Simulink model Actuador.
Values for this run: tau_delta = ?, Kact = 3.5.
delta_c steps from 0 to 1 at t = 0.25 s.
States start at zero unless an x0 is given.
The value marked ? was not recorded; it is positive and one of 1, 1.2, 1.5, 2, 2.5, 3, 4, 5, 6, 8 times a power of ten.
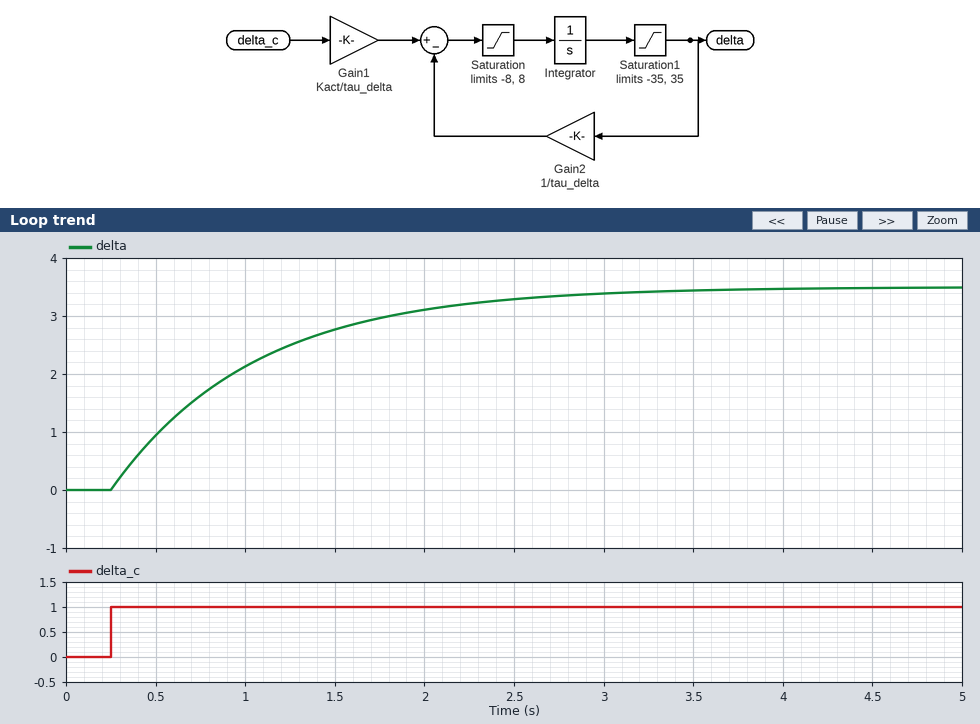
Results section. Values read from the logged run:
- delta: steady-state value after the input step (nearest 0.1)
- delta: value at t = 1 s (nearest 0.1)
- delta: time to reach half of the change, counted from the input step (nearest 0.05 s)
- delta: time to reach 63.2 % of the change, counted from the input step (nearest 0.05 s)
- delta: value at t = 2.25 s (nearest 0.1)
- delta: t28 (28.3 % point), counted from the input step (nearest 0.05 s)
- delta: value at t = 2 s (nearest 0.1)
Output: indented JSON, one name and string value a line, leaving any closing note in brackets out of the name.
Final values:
{
  "delta: steady-state value after the input step": "3.5",
  "delta: value at t = 1 s": "2.1",
  "delta: time to reach half of the change, counted from the input step": "0.55 s",
  "delta: time to reach 63.2 % of the change, counted from the input step": "0.80 s",
  "delta: value at t = 2.25 s": "3.2",
  "delta: t28 (28.3 % point), counted from the input step": "0.25 s",
  "delta: value at t = 2 s": "3.1"
}
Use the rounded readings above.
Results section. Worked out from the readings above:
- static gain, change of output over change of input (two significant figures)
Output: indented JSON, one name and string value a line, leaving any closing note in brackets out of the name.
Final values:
{
  "static gain, change of output over change of input": "3.5"
}
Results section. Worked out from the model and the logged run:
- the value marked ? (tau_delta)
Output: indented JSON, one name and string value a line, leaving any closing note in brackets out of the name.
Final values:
{
  "the value marked ?": "0.8"
}
